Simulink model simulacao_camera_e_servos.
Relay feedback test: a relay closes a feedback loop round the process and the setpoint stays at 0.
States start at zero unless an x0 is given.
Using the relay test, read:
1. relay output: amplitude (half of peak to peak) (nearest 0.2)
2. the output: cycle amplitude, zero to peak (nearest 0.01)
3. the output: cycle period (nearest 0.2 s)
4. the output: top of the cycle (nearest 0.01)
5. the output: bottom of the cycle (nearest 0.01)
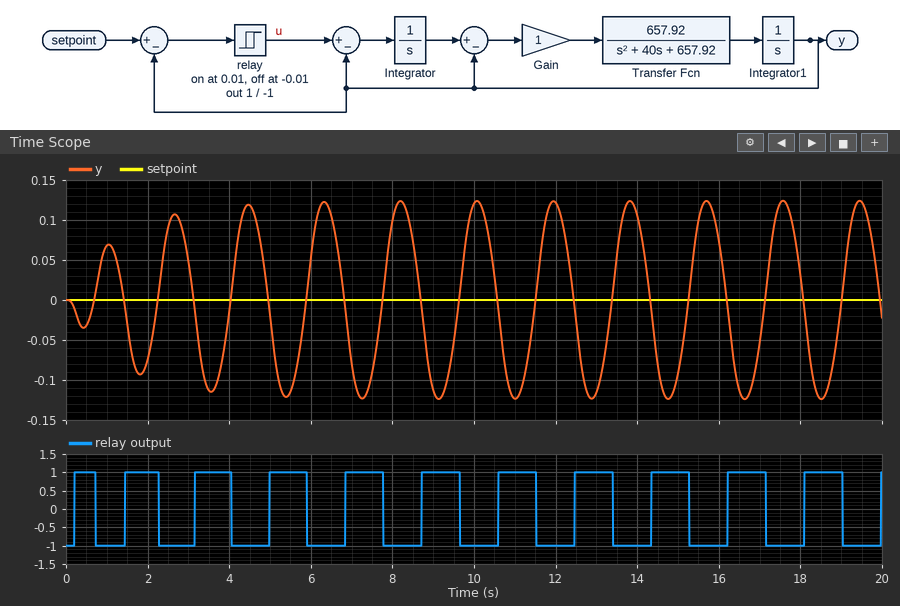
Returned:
1.0
0.12
1.8 s
0.12
-0.12
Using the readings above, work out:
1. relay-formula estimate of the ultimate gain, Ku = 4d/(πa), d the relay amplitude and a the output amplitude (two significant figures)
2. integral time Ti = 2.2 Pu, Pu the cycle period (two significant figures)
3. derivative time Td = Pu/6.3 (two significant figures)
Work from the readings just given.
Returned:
11
4.0 s
0.29 s
